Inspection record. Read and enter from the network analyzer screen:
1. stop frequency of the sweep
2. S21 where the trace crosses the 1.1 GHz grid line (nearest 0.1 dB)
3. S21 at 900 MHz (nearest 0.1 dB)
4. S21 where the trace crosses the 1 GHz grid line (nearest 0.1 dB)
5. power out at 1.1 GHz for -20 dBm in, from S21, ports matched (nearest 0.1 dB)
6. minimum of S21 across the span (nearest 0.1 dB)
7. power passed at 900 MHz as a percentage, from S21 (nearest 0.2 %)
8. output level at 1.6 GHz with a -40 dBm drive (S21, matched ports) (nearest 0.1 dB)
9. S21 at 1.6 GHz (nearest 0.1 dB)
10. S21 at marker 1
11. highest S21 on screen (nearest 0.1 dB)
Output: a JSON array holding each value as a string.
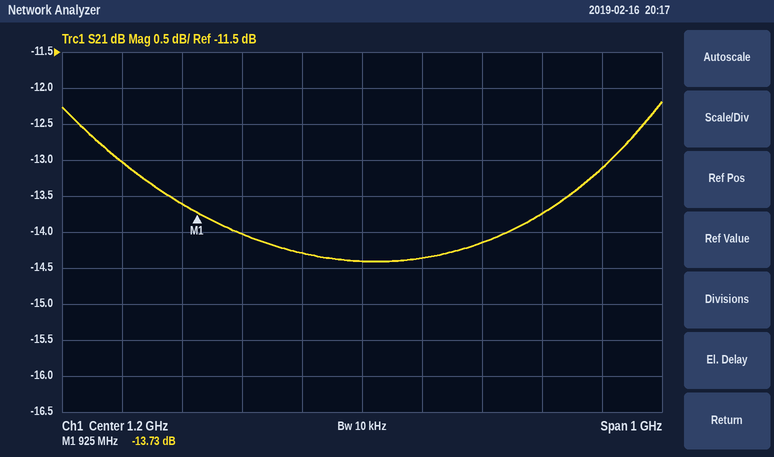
["1.7 GHz", "-14.3 dB", "-13.6 dB", "-14.0 dB", "-34.3 dBm", "-14.4 dB", "4.4 %", "-53.1 dBm", "-13.1 dB", "-13.73 dB", "-12.2 dB"]
